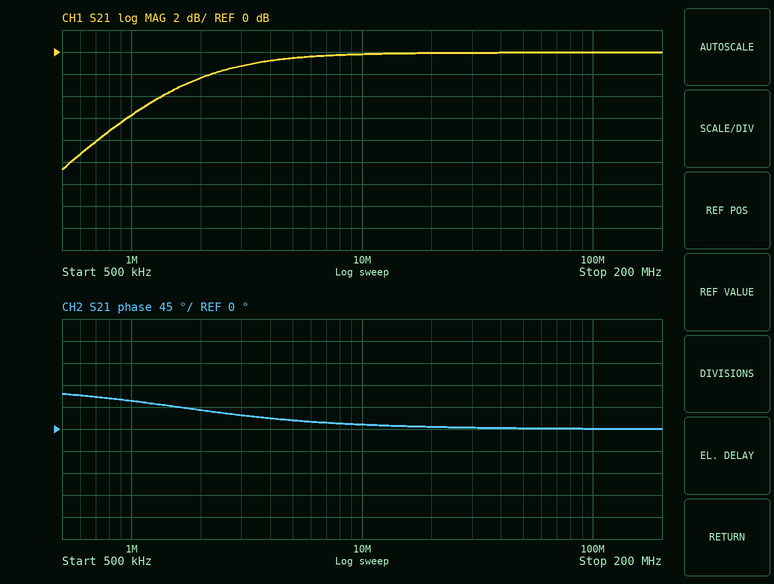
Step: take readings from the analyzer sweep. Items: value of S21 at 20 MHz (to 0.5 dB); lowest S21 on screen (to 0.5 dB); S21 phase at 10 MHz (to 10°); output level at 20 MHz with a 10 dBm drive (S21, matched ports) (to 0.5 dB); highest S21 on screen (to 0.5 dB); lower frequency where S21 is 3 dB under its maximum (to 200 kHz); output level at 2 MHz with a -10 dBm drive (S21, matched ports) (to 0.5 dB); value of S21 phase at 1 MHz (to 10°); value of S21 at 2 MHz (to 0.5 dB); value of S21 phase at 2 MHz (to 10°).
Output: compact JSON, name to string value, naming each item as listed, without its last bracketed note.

{"value of S21 at 20 MHz": "0.0 dB", "lowest S21 on screen": "-10.5 dB", "S21 phase at 10 MHz": "10°", "output level at 20 MHz with a 10 dBm drive (S21, matched ports)": "10.0 dBm", "highest S21 on screen": "0.0 dB", "lower frequency where S21 is 3 dB under its maximum": "1.6 MHz", "output level at 2 MHz with a -10 dBm drive (S21, matched ports)": "-12.5 dBm", "value of S21 phase at 1 MHz": "60°", "value of S21 at 2 MHz": "-2.5 dB", "value of S21 phase at 2 MHz": "40°"}
